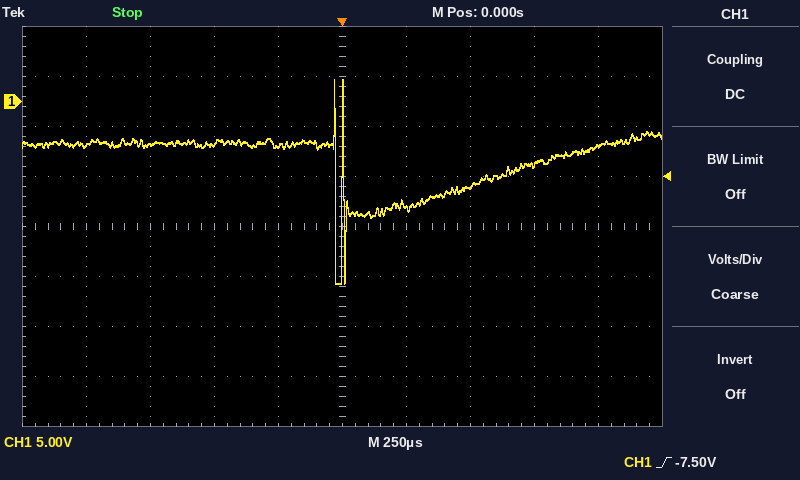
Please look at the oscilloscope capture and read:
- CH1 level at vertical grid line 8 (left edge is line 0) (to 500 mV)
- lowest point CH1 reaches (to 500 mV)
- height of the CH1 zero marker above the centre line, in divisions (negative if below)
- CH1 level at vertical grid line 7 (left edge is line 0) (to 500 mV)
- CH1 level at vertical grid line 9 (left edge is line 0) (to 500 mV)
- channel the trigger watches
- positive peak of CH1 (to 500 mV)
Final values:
-6.5 V
-18.0 V
+2.5 div
-8.5 V
-4.5 V
CH1
2.0 V
